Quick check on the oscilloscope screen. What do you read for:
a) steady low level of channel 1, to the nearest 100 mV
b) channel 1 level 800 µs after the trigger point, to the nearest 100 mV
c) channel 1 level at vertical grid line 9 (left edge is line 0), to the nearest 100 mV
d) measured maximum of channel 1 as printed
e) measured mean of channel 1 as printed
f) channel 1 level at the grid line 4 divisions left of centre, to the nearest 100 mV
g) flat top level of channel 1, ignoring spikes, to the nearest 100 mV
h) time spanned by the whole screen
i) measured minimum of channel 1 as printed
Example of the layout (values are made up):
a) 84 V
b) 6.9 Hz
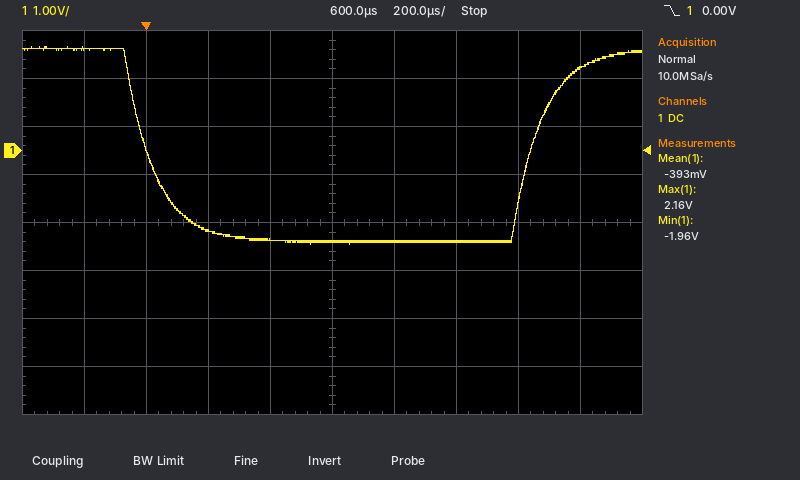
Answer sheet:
a) -1.9 V
b) -1.9 V
c) 1.7 V
d) 2.16 V
e) -393 mV
f) 2.1 V
g) 2.1 V
h) 2 ms
i) -1.96 V
